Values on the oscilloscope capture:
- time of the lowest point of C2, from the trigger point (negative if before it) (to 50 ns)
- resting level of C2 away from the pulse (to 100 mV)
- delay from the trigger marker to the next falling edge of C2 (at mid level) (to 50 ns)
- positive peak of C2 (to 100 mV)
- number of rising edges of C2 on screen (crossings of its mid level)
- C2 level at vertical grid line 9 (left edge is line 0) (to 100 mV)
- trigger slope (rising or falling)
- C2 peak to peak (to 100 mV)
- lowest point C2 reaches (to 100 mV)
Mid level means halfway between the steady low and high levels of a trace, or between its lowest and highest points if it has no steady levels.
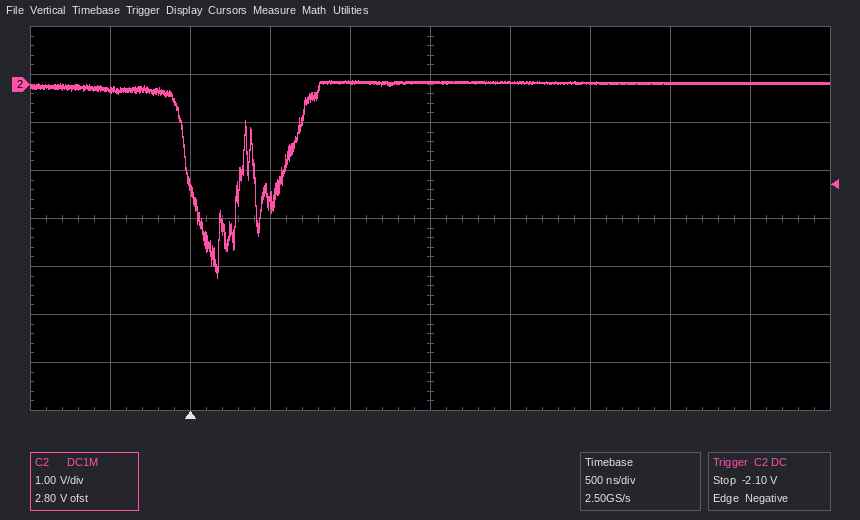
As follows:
+150 ns
0.0 V
400 ns
100 mV
2
0.0 V
falling
4.1 V
-4.0 V
